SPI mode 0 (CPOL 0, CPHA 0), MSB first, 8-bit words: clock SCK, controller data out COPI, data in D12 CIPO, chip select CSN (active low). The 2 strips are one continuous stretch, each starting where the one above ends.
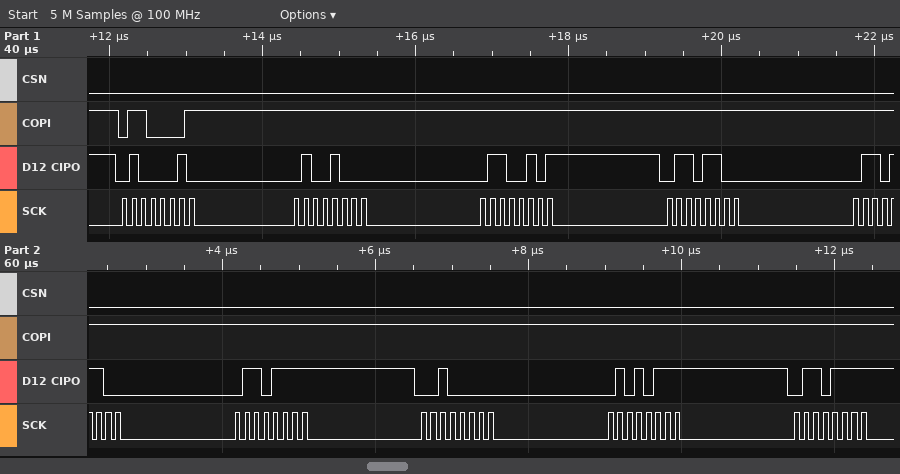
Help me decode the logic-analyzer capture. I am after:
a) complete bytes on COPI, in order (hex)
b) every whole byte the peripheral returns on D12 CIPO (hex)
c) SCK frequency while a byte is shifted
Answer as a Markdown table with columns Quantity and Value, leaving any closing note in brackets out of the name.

| Quantity | Value |
|---|---|
| complete bytes on COPI, in order | 61 FF FF FF FF FF FF FF FF |
| every whole byte the peripheral returns on D12 CIPO | 42 48 65 6C 6C 6F 20 57 6F |
| SCK frequency while a byte is shifted | 8 MHz |
